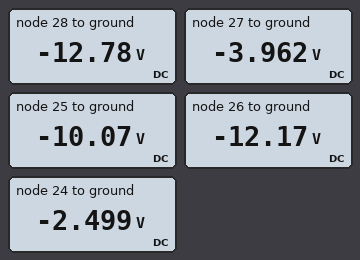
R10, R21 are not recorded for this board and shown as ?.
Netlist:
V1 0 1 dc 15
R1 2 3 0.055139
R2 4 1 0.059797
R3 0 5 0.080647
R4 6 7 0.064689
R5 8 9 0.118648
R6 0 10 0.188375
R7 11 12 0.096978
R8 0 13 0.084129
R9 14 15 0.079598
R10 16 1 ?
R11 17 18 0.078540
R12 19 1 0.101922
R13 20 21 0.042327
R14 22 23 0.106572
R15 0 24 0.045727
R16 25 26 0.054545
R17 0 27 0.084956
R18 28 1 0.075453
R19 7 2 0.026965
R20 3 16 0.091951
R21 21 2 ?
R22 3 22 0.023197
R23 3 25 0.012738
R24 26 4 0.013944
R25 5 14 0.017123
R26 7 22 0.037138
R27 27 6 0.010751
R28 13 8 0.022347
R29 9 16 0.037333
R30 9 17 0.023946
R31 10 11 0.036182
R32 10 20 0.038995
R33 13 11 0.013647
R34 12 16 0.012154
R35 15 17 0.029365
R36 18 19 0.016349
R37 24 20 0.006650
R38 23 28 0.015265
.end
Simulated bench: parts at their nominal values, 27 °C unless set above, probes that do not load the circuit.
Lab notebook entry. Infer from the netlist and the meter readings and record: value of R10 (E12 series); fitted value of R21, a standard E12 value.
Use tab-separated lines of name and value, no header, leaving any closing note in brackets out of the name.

value of R10	0.033 Ω
fitted value of R21, a standard E12 value	0.082 Ω
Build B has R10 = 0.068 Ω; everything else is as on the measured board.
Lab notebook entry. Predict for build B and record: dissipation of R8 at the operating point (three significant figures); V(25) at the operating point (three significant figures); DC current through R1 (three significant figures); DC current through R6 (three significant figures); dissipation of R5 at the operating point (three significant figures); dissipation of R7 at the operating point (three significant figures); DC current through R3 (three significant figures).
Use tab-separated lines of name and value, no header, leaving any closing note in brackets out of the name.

dissipation of R8 at the operating point	184 W
V(25) at the operating point	-9.48 V
DC current through R1	35.1 A
DC current through R6	16.4 A
dissipation of R5 at the operating point	103 W
dissipation of R7 at the operating point	215 W
DC current through R3	38.7 A
